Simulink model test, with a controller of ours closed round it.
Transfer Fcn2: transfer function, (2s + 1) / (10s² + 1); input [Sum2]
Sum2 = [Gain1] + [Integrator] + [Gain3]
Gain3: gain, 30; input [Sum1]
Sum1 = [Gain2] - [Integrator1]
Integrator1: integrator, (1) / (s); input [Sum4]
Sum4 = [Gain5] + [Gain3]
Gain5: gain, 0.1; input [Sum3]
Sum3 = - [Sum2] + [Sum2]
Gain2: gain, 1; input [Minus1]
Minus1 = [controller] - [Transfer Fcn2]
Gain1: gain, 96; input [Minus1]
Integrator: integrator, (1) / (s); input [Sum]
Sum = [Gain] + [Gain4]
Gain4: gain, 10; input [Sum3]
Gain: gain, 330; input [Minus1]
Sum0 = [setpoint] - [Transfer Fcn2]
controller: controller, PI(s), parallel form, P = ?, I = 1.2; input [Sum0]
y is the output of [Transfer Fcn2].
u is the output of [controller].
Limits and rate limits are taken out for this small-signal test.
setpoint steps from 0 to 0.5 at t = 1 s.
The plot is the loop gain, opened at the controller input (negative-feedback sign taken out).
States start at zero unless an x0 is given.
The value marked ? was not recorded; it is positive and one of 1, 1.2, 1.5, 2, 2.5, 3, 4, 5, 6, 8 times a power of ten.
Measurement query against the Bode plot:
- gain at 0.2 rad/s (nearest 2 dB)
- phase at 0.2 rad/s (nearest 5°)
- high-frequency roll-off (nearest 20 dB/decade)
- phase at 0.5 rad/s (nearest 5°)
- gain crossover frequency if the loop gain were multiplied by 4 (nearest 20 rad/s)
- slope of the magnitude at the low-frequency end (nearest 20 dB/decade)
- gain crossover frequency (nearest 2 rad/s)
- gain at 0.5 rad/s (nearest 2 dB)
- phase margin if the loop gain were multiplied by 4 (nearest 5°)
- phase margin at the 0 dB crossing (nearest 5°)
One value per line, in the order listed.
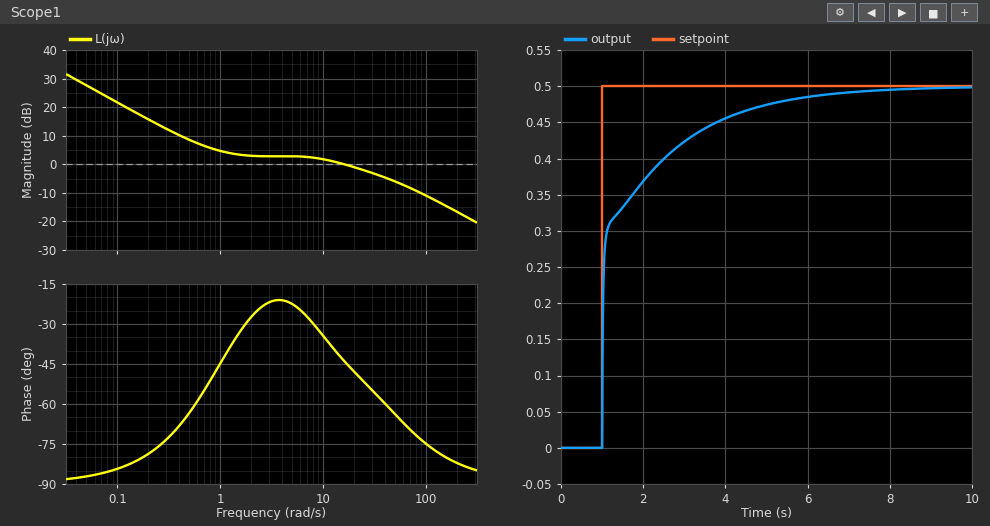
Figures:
16 dB
-80°
-20 dB/decade
-65°
120 rad/s
-20 dB/decade
16 rad/s
8 dB
105°
135°
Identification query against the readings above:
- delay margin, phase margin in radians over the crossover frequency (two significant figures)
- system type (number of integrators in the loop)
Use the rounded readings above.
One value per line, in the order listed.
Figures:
0.15 s
1
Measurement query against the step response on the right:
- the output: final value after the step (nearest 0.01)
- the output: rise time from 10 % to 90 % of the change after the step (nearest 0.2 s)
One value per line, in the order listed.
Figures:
0.50
2.8 s
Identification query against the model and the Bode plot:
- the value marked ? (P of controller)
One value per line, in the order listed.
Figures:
1.2
